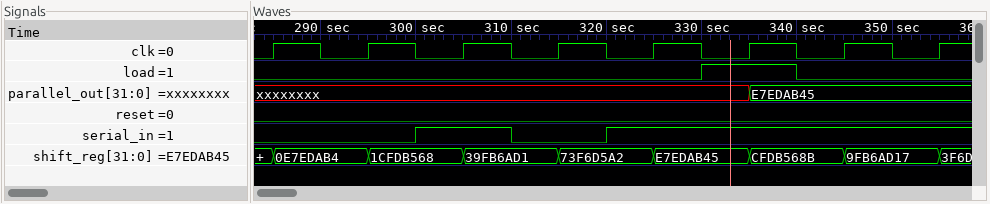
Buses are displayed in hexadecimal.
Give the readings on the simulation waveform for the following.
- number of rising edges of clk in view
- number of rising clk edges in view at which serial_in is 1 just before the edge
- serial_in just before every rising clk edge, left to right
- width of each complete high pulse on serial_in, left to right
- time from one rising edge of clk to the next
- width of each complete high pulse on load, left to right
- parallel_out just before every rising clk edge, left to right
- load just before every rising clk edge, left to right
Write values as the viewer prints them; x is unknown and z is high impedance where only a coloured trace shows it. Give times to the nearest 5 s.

8
5
0 0 1 0 1 1 1 1
10 s
10 s
10 s
xxxxxxxx, xxxxxxxx, xxxxxxxx, xxxxxxxx, xxxxxxxx, xxxxxxxx, E7EDAB45, E7EDAB45
0 0 0 0 0 1 0 0
